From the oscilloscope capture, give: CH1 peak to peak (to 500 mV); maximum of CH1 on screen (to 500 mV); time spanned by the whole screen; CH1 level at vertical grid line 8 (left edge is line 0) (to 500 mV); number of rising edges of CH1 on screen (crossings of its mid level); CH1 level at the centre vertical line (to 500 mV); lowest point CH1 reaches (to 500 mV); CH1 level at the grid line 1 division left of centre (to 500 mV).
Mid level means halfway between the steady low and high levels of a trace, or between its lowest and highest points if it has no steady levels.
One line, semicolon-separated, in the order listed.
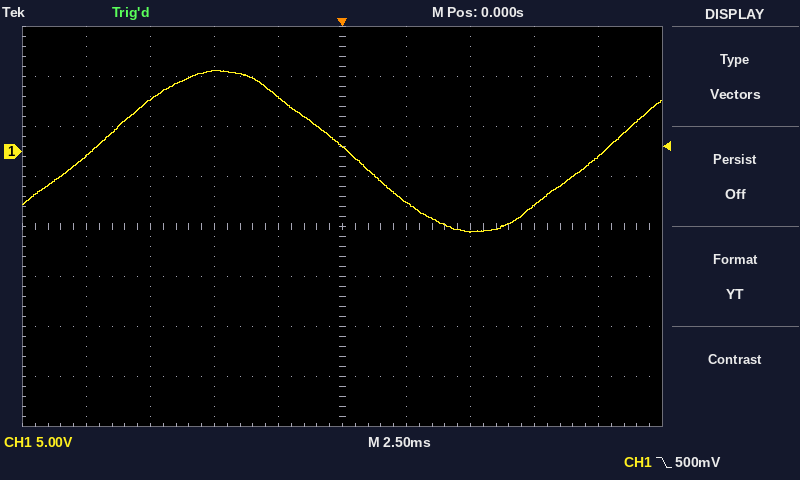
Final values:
16.0 V; 8.0 V; 25 ms; -5.5 V; 2; 500 mV; -8.0 V; 5.5 V
